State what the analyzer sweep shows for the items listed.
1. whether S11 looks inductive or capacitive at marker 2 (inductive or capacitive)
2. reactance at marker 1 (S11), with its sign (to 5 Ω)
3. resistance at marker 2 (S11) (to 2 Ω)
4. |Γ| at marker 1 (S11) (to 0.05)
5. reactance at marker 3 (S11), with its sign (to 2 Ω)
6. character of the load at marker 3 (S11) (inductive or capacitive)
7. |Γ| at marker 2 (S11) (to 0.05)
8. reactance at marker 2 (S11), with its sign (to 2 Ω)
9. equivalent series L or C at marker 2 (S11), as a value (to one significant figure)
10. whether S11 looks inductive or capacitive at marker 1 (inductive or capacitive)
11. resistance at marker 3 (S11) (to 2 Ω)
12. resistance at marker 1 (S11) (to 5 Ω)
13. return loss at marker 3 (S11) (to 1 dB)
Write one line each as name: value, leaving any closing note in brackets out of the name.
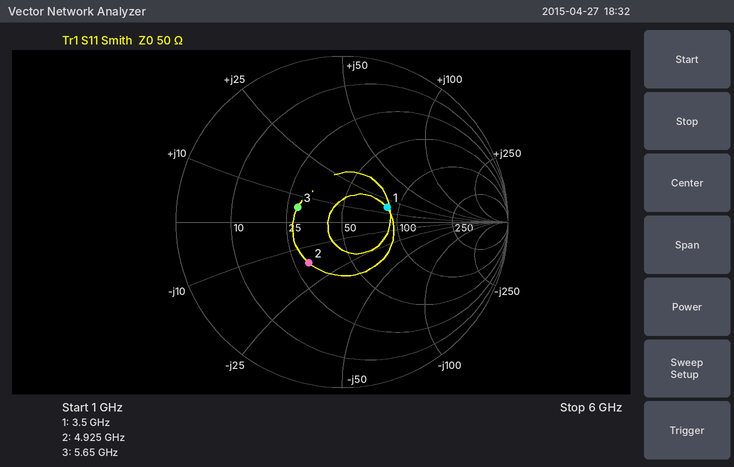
whether S11 looks inductive or capacitive at marker 2: capacitive
reactance at marker 1 (S11), with its sign: +15 Ω
resistance at marker 2 (S11): 30 Ω
|Γ| at marker 1 (S11): 0.30
reactance at marker 3 (S11), with its sign: +6 Ω
character of the load at marker 3 (S11): inductive
|Γ| at marker 2 (S11): 0.30
reactance at marker 2 (S11), with its sign: -16 Ω
equivalent series L or C at marker 2 (S11), as a value: 2 pF
whether S11 looks inductive or capacitive at marker 1: inductive
resistance at marker 3 (S11): 28 Ω
resistance at marker 1 (S11): 85 Ω
return loss at marker 3 (S11): 11 dB
